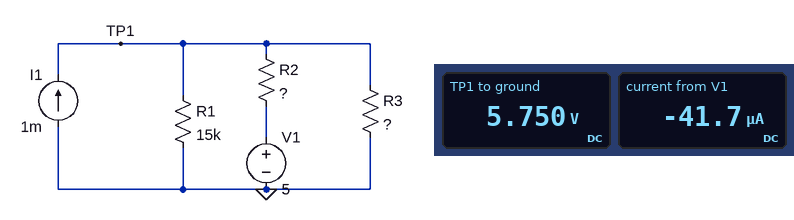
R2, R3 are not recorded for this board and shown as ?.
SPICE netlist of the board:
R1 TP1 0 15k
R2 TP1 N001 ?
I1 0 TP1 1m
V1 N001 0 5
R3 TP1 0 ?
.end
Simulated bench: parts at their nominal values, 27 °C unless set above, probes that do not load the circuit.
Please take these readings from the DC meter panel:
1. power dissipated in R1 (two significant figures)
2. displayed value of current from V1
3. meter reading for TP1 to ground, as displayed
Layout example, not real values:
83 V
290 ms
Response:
2.2 mW
-41.7 µA
5.750 V
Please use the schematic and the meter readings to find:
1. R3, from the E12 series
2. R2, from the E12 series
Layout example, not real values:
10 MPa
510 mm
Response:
10 kΩ
18 kΩ
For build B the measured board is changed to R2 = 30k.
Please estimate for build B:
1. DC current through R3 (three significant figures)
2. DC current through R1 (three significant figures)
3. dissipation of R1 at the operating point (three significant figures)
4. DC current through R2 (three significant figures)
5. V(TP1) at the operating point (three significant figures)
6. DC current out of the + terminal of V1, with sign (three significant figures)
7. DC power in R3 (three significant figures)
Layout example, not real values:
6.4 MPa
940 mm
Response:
583 µA
389 µA
2.27 mW
27.8 µA
5.83 V
-27.8 µA
3.40 mW
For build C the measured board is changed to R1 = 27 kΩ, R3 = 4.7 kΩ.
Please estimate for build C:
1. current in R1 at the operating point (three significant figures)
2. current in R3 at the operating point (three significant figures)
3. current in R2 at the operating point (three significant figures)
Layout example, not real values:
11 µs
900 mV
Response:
155 µA
890 µA
45.3 µA
